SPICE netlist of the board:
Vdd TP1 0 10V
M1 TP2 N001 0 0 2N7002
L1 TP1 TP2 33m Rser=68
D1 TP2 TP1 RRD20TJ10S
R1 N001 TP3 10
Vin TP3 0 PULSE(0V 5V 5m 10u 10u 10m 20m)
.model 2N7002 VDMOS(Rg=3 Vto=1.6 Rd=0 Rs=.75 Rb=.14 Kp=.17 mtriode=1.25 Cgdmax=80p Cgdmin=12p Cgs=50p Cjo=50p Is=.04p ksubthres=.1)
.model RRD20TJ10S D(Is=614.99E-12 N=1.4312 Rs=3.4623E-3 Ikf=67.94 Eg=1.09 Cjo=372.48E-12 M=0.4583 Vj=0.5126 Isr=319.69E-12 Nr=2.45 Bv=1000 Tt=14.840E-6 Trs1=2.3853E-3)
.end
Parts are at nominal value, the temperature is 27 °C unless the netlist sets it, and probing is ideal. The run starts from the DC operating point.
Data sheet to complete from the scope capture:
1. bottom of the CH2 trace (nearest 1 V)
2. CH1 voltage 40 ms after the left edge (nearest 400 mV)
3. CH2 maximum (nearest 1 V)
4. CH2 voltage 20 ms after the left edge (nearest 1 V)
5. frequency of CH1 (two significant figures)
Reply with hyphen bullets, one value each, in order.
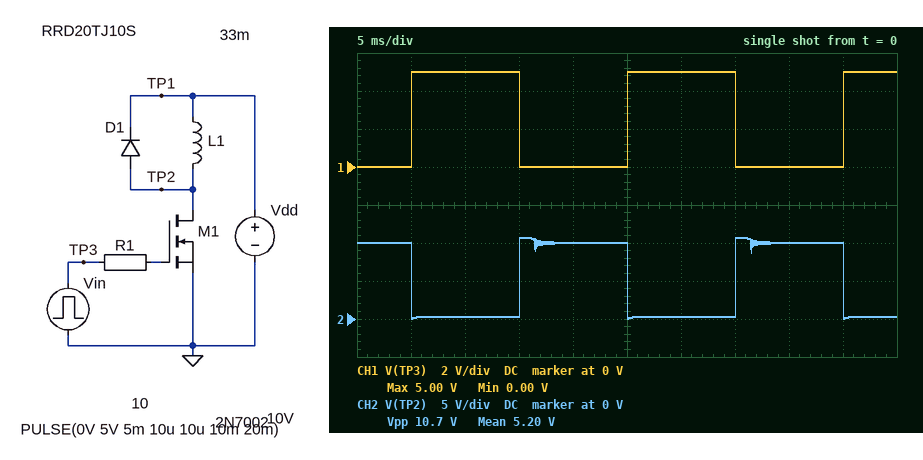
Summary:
- 0 V
- 0 V
- 11 V
- 10 V
- 50 Hz
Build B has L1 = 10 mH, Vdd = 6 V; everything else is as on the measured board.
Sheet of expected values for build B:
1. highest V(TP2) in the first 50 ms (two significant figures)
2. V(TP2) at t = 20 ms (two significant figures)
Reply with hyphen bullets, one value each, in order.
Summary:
- 6.7 V
- 6.0 V
